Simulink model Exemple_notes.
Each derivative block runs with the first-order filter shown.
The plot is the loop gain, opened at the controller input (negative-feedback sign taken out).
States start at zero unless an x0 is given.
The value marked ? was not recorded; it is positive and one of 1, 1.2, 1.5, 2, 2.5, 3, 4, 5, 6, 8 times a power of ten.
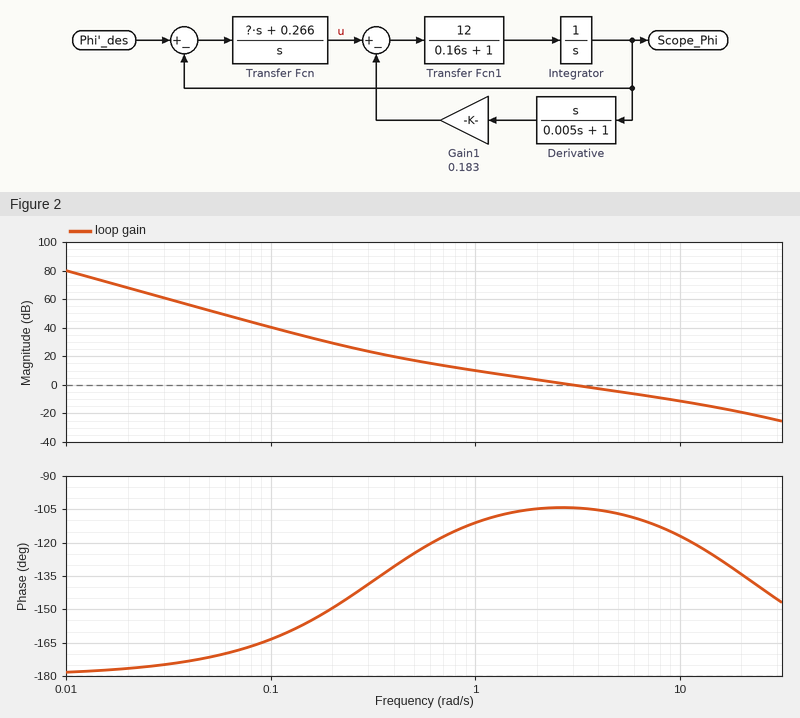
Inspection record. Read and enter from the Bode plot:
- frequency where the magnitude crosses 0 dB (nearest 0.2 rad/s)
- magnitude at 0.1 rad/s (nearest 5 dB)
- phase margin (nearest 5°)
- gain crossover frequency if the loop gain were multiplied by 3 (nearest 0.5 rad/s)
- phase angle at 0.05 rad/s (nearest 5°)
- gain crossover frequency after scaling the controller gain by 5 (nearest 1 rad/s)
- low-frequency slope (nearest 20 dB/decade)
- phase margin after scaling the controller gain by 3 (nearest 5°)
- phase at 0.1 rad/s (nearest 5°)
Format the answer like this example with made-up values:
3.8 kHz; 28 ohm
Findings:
3.0 rad/s; 40 dB; 75°; 8.5 rad/s; -170°; 13 rad/s; -40 dB/decade; 65°; -165°
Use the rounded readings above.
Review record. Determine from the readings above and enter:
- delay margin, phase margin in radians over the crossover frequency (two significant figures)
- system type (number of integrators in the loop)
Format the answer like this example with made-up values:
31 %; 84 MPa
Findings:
0.44 s; 2
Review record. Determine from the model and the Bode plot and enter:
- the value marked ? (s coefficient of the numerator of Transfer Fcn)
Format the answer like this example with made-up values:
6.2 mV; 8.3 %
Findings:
0.8
